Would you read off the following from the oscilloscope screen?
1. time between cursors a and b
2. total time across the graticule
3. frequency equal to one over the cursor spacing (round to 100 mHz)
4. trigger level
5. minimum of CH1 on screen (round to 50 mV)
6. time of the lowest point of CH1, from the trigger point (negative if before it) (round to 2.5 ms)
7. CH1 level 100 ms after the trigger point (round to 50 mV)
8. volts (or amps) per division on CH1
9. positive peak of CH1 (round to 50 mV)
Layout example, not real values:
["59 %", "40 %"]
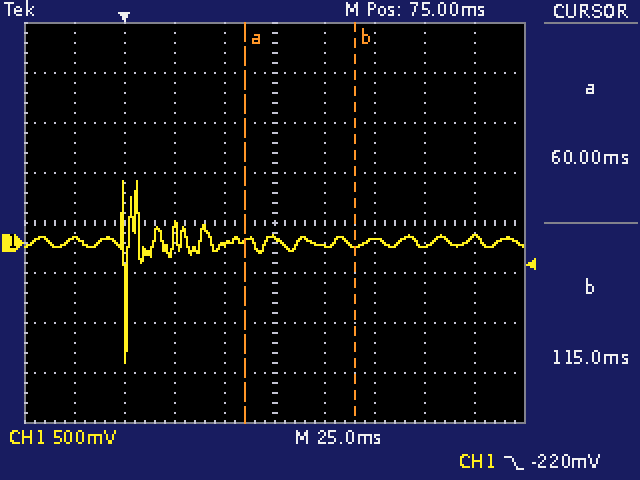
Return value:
["55.0 ms", "250 ms", "18.2 Hz", "-220 mV", "-1.20 V", "0.0 ms", "-50 mV", "500 mV", "600 mV"]
